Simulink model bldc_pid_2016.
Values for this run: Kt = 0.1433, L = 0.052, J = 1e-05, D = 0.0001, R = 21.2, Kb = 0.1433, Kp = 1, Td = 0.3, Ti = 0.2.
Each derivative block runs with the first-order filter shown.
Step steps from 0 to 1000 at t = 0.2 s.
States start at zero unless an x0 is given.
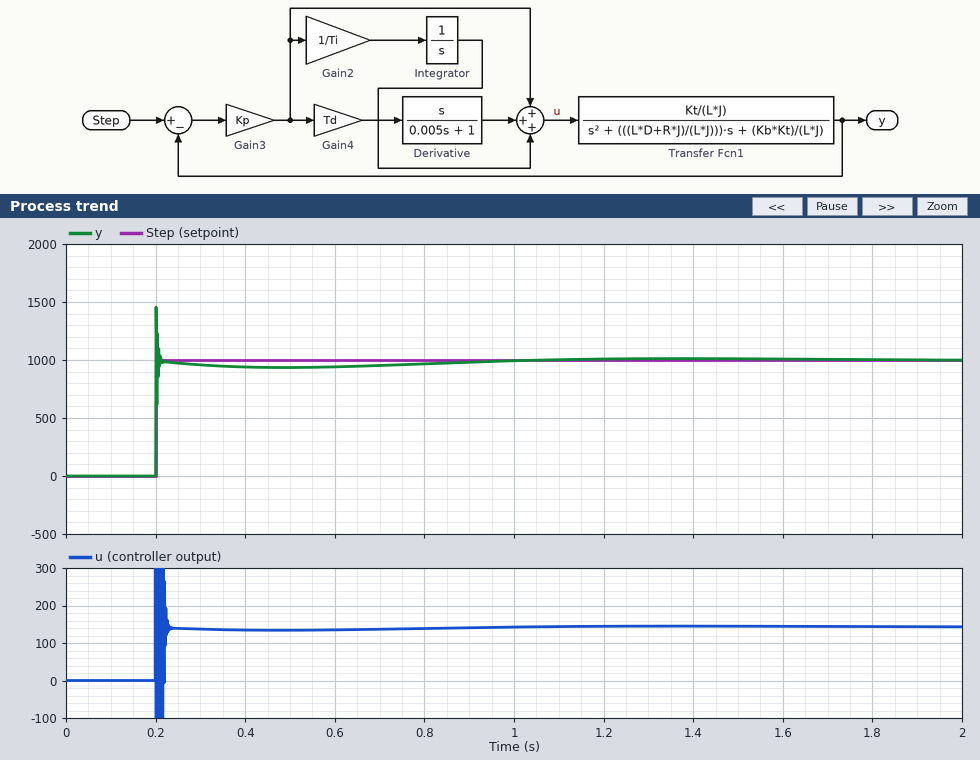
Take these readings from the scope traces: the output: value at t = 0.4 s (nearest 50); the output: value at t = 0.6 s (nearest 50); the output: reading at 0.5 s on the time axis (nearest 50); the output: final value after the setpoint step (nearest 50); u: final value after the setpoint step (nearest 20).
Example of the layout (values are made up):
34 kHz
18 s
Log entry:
950
950
950
1000
140
